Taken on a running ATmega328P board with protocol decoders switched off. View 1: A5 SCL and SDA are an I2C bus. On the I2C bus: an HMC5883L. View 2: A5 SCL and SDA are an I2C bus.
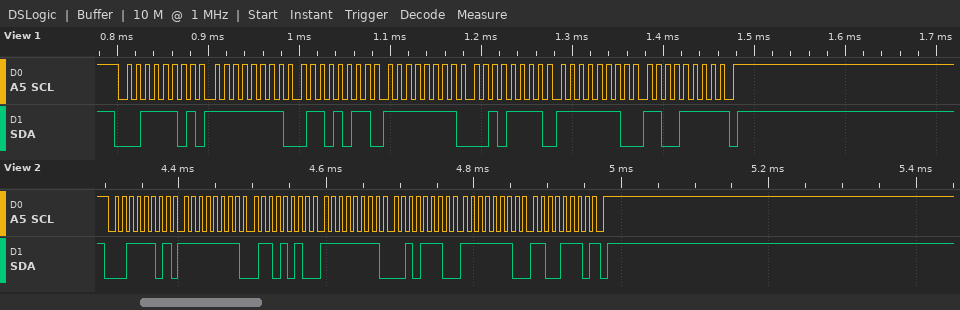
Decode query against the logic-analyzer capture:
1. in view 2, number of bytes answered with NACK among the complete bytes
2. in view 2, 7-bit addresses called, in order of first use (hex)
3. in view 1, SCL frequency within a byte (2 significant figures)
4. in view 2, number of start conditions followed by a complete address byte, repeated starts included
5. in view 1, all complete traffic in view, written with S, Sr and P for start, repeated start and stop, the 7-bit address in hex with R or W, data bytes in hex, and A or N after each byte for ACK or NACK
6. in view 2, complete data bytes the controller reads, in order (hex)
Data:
1
0x1E
100 kHz
1
S 1ER A FF A 6B A FF A 2F A FE A CF N P
FF 6A FF 2E FE CE
